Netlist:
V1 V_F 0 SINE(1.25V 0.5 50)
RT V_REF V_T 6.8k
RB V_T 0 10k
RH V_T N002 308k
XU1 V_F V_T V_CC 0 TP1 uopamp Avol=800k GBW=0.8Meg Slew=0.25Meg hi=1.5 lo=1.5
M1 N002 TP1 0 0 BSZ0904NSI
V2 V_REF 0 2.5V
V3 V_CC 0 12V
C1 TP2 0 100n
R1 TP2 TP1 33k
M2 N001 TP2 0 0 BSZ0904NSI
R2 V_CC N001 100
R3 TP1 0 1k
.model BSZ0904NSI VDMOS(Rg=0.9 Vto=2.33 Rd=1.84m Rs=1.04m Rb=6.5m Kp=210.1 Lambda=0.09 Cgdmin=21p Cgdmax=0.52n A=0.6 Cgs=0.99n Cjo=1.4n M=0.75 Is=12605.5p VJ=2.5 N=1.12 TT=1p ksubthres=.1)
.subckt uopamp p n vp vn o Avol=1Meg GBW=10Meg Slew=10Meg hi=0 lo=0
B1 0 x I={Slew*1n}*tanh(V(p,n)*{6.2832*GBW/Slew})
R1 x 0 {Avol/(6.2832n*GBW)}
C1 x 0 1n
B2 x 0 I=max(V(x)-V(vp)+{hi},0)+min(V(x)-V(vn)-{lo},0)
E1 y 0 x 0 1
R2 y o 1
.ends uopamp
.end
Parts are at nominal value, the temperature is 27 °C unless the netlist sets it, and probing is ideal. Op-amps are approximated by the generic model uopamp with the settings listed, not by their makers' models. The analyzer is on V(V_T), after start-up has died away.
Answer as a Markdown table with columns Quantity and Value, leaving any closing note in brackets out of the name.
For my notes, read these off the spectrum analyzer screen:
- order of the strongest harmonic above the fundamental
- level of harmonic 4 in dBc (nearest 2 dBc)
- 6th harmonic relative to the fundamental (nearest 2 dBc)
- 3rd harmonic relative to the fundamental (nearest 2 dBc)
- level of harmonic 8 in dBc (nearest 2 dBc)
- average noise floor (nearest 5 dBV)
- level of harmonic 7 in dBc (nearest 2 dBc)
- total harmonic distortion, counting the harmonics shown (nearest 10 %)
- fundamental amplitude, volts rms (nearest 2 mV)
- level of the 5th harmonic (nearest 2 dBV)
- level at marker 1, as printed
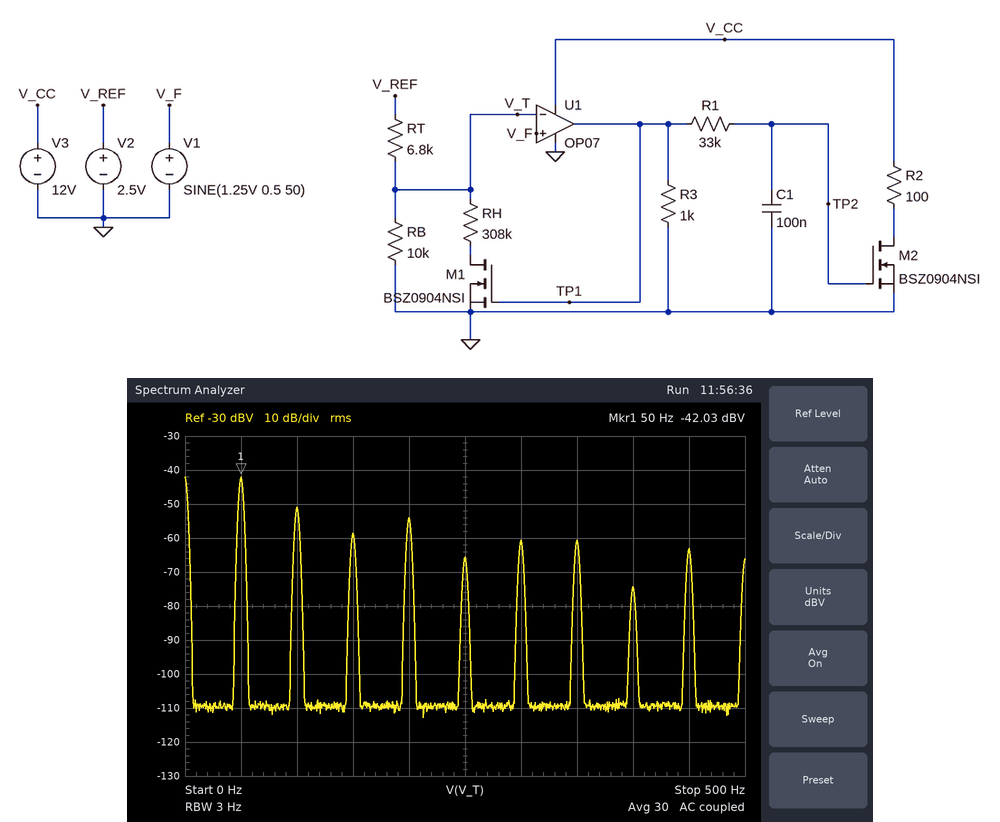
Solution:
| Quantity | Value |
|---|---|
| order of the strongest harmonic above the fundamental | 2 |
| level of harmonic 4 in dBc | -12 dBc |
| 6th harmonic relative to the fundamental | -18 dBc |
| 3rd harmonic relative to the fundamental | -16 dBc |
| level of harmonic 8 in dBc | -32 dBc |
| average noise floor | -110 dBV |
| level of harmonic 7 in dBc | -18 dBc |
| total harmonic distortion, counting the harmonics shown | 50 % |
| fundamental amplitude, volts rms | 8 mV |
| level of the 5th harmonic | -66 dBV |
| level at marker 1, as printed | -42.03 dBV |
